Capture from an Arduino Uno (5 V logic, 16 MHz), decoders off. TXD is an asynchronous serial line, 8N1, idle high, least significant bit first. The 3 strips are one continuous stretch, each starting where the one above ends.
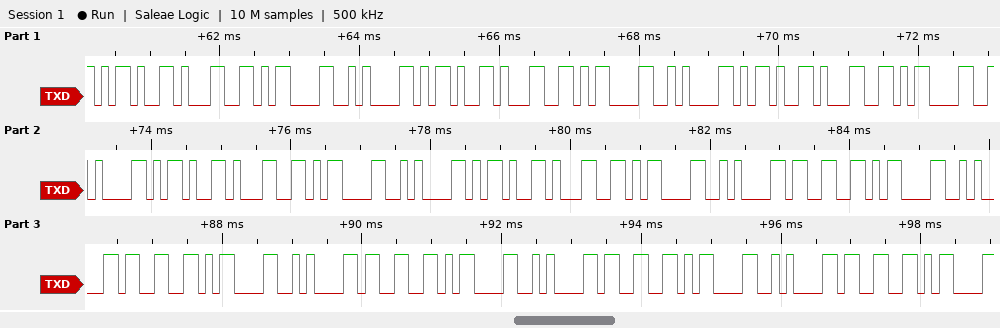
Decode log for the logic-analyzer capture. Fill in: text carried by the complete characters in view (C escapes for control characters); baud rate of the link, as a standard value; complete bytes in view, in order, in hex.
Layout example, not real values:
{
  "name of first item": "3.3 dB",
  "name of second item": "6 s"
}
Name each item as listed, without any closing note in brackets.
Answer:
{
  "text carried by the complete characters in view": "\"-1\\r\\n-1\\r\\n-1\\r\\n-1\\r\\n-1\\r\\n3\\r\\n3\\r\\n3\\r\\n3\\r\\n3\\r\"",
  "baud rate of the link, as a standard value": "9600 baud",
  "complete bytes in view, in order, in hex": "2D 31 0D 0A 2D 31 0D 0A 2D 31 0D 0A 2D 31 0D 0A 2D 31 0D 0A 33 0D 0A 33 0D 0A 33 0D 0A 33 0D 0A 33 0D"
}
